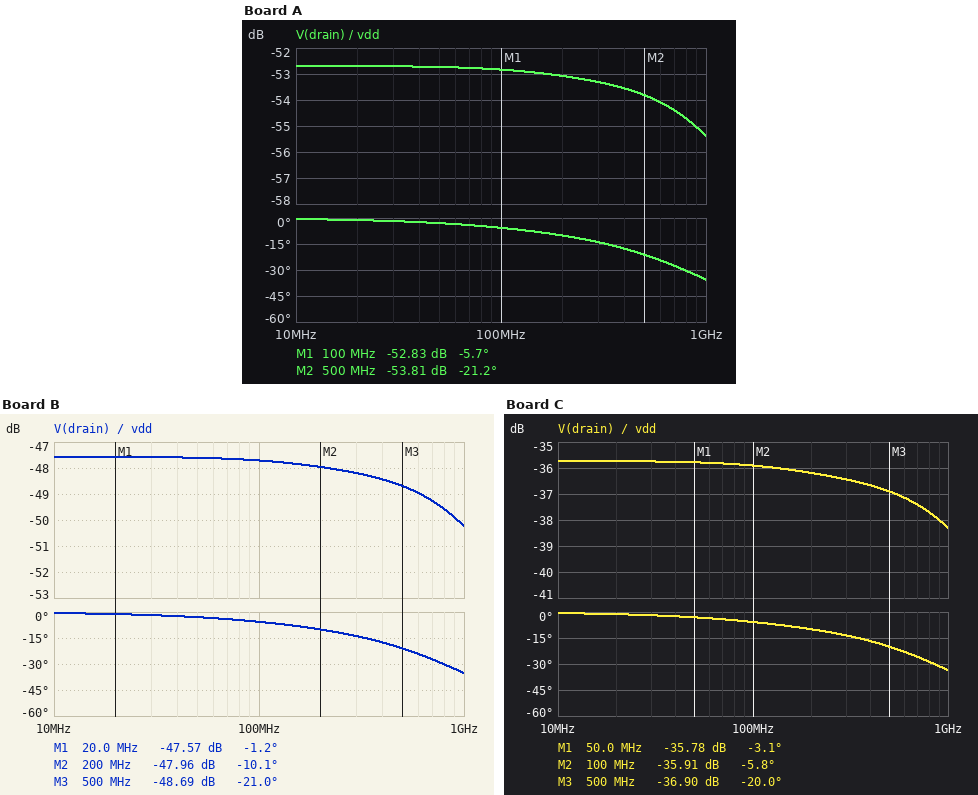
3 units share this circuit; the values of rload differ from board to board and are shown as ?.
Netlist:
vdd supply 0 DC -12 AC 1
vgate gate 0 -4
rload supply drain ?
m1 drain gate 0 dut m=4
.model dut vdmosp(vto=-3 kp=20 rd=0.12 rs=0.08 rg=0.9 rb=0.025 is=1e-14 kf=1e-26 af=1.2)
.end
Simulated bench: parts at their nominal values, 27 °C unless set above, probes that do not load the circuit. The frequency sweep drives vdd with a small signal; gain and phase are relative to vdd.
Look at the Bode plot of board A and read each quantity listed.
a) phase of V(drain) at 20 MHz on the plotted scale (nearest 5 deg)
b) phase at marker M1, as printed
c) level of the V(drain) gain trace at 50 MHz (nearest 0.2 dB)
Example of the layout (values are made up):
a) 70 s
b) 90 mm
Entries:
a) 0 deg
b) -5.7 deg
c) -52.8 dB
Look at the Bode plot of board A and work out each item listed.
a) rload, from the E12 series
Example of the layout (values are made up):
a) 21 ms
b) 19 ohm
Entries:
a) 27 Ω
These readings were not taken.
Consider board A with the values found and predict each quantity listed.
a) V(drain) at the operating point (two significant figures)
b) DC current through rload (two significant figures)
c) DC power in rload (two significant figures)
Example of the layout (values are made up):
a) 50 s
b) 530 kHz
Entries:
a) -28 mV
b) 440 mA
c) 5.3 W
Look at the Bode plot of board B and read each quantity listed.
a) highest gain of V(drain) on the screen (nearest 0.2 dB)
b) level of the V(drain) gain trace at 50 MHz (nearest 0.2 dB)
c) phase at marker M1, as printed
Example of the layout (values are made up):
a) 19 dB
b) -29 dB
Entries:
a) -47.6 dB
b) -47.6 dB
c) -1.2 deg
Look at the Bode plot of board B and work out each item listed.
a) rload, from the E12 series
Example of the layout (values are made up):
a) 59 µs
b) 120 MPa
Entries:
a) 15 Ω
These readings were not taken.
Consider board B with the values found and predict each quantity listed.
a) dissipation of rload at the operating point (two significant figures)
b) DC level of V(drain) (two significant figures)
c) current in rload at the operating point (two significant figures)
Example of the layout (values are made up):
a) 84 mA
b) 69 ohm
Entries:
a) 9.5 W
b) -50 mV
c) 800 mA
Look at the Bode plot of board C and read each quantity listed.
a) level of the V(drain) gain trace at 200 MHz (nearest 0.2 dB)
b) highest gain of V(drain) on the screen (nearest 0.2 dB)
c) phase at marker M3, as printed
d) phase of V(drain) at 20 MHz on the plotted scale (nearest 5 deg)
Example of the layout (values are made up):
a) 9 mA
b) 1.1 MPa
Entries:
a) -36.2 dB
b) -35.8 dB
c) -20.0 deg
d) 0 deg
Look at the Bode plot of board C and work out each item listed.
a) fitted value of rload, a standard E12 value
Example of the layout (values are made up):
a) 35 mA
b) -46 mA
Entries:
a) 3.9 Ω
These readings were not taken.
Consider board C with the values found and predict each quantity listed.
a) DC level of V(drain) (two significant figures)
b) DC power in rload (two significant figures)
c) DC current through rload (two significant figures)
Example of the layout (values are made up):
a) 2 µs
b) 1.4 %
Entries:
a) -190 mV
b) 36 W
c) 3.0 A
